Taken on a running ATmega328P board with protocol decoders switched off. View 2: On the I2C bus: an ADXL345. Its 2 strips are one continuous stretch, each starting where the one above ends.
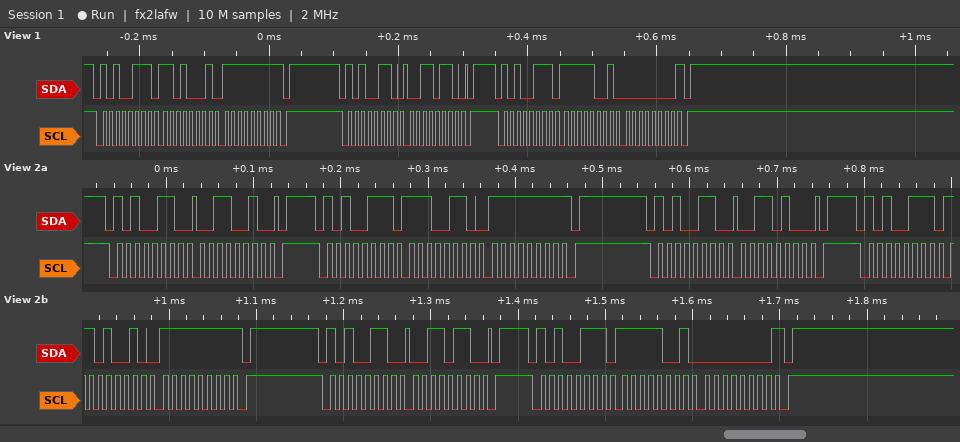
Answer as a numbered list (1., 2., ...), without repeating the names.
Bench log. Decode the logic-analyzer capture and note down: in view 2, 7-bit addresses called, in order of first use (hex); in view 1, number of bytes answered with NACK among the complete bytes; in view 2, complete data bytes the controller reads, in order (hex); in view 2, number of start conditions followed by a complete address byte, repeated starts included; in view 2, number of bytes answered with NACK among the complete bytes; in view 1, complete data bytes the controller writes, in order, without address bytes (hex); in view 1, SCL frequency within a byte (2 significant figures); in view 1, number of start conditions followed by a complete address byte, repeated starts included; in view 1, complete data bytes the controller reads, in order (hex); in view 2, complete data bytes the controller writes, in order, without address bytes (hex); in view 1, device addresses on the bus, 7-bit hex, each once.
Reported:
1. 0x53
2. 2
3. E6 FF D2 FF F9 00
4. 6
5. 3
6. 36
7. 100 kHz
8. 3
9. D1 FF F9 00
10. 32 34 36
11. 0x53
